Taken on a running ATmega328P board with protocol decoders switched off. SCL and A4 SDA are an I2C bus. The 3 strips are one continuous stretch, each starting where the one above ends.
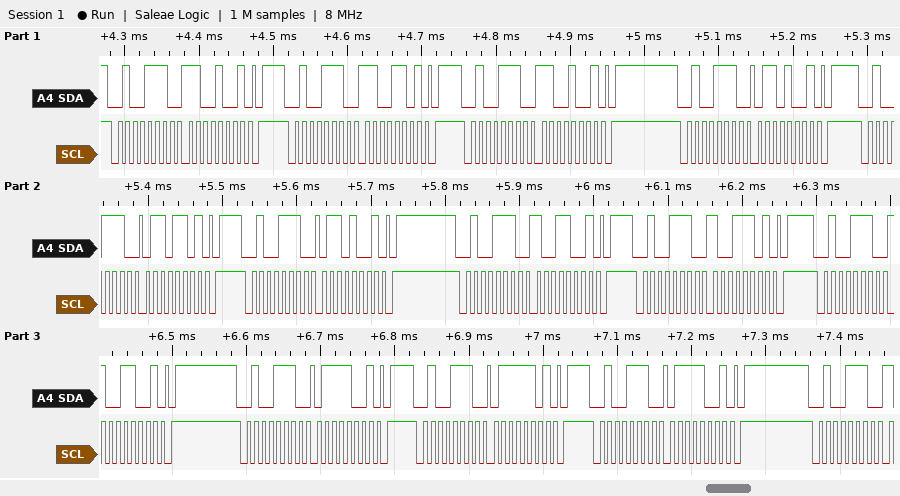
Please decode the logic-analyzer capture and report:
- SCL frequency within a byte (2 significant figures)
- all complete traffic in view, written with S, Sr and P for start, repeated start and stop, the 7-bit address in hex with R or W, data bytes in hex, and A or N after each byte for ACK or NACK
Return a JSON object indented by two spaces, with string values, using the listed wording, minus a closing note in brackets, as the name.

{
  "SCL frequency within a byte": "100 kHz",
  "all complete traffic in view, written with S, Sr and P for start, repeated start and stop, the 7-bit address in hex with R or W, data bytes in hex, and A or N after each byte for ACK or NACK": "S 27W A C9 A P S 27W A CD A P S 27W A C9 A P S 27W A 69 A P S 27W A 6D A P S 27W A 69 A P S 27W A 99 A P S 27W A 9D A P S 27W A 99 A P S 27W A 79 A P S 27W A 7D A P S 27W A 79 A P S 27W A"
}
